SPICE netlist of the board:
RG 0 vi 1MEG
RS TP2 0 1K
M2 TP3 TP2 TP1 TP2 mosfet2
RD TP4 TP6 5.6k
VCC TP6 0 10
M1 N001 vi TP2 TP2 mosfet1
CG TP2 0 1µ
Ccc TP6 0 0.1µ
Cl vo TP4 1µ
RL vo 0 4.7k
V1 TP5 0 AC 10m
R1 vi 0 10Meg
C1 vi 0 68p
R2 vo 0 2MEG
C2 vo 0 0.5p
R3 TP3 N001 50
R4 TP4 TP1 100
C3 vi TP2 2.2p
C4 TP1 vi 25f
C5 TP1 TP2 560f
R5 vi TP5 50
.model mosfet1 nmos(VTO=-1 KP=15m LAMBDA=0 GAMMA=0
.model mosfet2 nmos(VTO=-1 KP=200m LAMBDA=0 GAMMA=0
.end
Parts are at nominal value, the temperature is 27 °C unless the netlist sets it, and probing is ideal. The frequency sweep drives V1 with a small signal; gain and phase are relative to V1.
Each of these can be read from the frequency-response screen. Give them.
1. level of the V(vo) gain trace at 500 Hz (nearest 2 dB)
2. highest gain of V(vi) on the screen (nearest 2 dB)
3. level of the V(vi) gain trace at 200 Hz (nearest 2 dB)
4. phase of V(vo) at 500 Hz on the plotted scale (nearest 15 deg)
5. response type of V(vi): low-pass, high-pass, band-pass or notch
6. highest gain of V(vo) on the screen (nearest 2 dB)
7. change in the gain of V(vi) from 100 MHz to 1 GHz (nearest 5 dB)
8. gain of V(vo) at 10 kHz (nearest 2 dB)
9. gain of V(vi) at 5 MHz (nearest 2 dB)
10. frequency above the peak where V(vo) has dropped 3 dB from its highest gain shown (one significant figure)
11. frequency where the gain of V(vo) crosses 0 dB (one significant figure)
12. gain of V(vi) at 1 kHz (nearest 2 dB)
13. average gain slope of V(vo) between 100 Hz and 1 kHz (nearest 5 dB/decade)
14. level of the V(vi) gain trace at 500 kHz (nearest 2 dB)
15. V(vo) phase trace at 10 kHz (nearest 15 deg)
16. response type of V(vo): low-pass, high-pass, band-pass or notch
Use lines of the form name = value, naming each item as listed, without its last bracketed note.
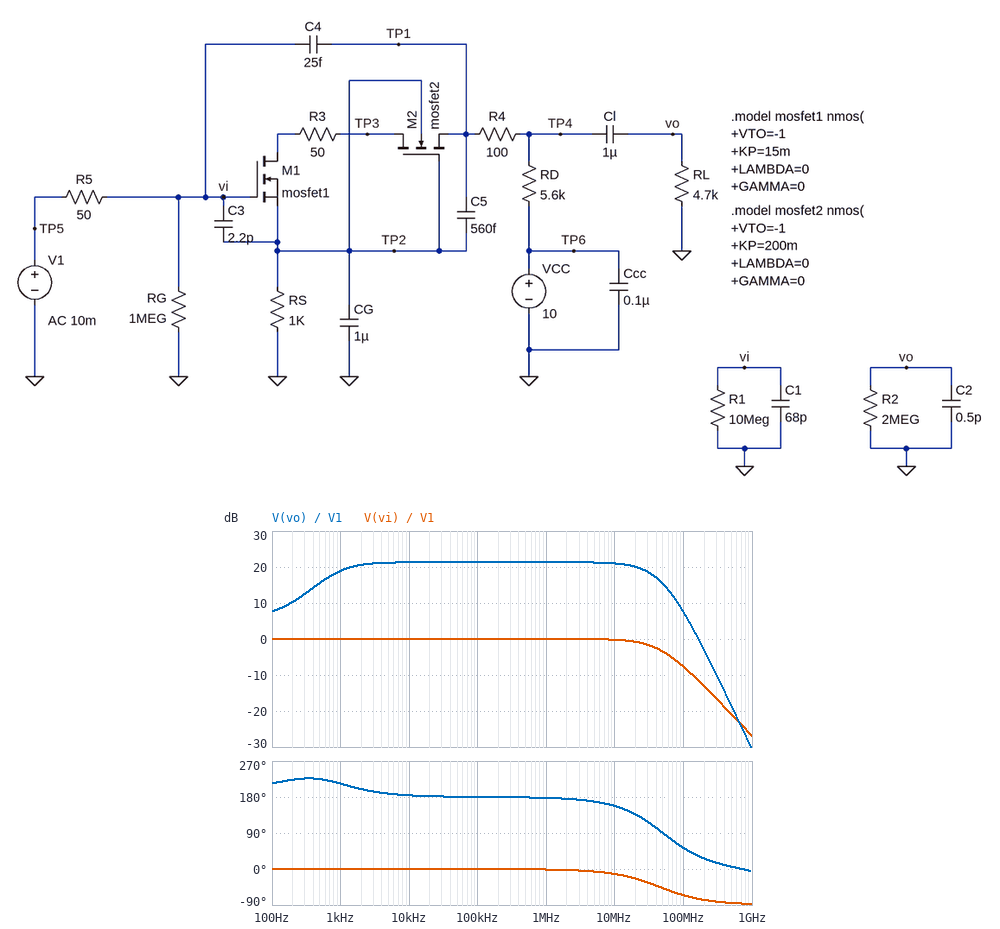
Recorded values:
level of the V(vo) gain trace at 500 Hz = 16 dB
highest gain of V(vi) on the screen = 0 dB
level of the V(vi) gain trace at 200 Hz = 0 dB
phase of V(vo) at 500 Hz on the plotted scale = 225 deg
response type of V(vi): low-pass, high-pass, band-pass or notch = low-pass
highest gain of V(vo) on the screen = 22 dB
change in the gain of V(vi) from 100 MHz to 1 GHz = -20 dB
gain of V(vo) at 10 kHz = 22 dB
gain of V(vi) at 5 MHz = 0 dB
frequency above the peak where V(vo) has dropped 3 dB from its highest gain shown = 30 MHz
frequency where the gain of V(vo) crosses 0 dB = 200 MHz
gain of V(vi) at 1 kHz = 0 dB
average gain slope of V(vo) between 100 Hz and 1 kHz = 10 dB/decade
level of the V(vi) gain trace at 500 kHz = 0 dB
V(vo) phase trace at 10 kHz = 180 deg
response type of V(vo): low-pass, high-pass, band-pass or notch = band-pass
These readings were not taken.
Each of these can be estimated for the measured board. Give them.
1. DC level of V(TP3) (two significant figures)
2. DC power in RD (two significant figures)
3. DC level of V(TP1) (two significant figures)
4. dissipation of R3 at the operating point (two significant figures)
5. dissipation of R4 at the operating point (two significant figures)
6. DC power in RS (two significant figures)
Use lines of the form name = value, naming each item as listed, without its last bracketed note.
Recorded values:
DC level of V(TP3) = 1.6 V
DC power in RD = 2.7 mW
DC level of V(TP1) = 6.0 V
dissipation of R3 at the operating point = 24 µW
dissipation of R4 at the operating point = 48 µW
DC power in RS = 480 µW
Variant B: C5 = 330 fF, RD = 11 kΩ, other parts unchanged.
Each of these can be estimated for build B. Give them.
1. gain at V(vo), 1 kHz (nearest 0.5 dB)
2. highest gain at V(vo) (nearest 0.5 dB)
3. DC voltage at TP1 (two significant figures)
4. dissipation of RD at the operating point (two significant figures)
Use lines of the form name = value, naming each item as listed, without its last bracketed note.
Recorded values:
gain at V(vo), 1 kHz = 21.0 dB
highest gain at V(vo) = 23.5 dB
DC voltage at TP1 = 2.3 V
dissipation of RD at the operating point = 5.3 mW
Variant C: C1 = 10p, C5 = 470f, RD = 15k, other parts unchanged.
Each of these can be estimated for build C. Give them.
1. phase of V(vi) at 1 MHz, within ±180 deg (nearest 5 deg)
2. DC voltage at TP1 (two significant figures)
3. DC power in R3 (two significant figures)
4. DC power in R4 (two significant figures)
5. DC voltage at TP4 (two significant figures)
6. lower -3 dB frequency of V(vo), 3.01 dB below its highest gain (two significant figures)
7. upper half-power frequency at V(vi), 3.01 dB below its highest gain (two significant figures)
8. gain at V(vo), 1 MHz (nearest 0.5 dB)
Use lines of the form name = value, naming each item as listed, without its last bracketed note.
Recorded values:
phase of V(vi) at 1 MHz, within ±180 deg = 0 deg
DC voltage at TP1 = 770 mV
DC power in R3 = 19 µW
DC power in R4 = 37 µW
DC voltage at TP4 = 830 mV
lower -3 dB frequency of V(vo), 3.01 dB below its highest gain = 76 Hz
upper half-power frequency at V(vi), 3.01 dB below its highest gain = 260 MHz
gain at V(vo), 1 MHz = -7.5 dB
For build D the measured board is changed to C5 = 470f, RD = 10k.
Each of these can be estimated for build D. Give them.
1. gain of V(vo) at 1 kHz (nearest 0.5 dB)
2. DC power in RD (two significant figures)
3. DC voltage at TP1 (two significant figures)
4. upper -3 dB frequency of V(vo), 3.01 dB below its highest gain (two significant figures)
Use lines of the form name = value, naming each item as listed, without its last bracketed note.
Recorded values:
gain of V(vo) at 1 kHz = 21.0 dB
DC power in RD = 4.8 mW
DC voltage at TP1 = 3.0 V
upper -3 dB frequency of V(vo), 3.01 dB below its highest gain = 30 MHz
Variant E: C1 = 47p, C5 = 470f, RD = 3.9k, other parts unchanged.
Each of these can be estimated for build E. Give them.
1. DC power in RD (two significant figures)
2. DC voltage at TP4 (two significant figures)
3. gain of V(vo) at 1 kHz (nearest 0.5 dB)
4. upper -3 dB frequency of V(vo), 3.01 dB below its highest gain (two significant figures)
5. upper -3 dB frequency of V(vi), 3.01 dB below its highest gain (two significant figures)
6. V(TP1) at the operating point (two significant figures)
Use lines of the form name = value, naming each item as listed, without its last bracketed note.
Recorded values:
DC power in RD = 1.9 mW
DC voltage at TP4 = 7.3 V
gain of V(vo) at 1 kHz = 17.5 dB
upper -3 dB frequency of V(vo), 3.01 dB below its highest gain = 44 MHz
upper -3 dB frequency of V(vi), 3.01 dB below its highest gain = 64 MHz
V(TP1) at the operating point = 7.2 V
